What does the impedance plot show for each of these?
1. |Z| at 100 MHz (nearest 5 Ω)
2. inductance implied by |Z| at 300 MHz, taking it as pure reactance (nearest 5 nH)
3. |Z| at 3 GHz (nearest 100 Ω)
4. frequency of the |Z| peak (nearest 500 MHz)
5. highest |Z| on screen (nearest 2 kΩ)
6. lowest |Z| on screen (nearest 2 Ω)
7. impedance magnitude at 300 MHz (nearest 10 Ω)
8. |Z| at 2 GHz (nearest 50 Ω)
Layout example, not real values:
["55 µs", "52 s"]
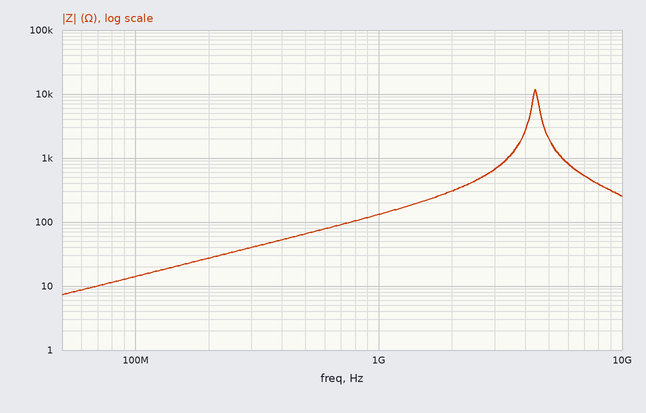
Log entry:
["15 Ω", "20 nH", "700 Ω", "4.5 GHz", "12 kΩ", "8 Ω", "40 Ω", "300 Ω"]
